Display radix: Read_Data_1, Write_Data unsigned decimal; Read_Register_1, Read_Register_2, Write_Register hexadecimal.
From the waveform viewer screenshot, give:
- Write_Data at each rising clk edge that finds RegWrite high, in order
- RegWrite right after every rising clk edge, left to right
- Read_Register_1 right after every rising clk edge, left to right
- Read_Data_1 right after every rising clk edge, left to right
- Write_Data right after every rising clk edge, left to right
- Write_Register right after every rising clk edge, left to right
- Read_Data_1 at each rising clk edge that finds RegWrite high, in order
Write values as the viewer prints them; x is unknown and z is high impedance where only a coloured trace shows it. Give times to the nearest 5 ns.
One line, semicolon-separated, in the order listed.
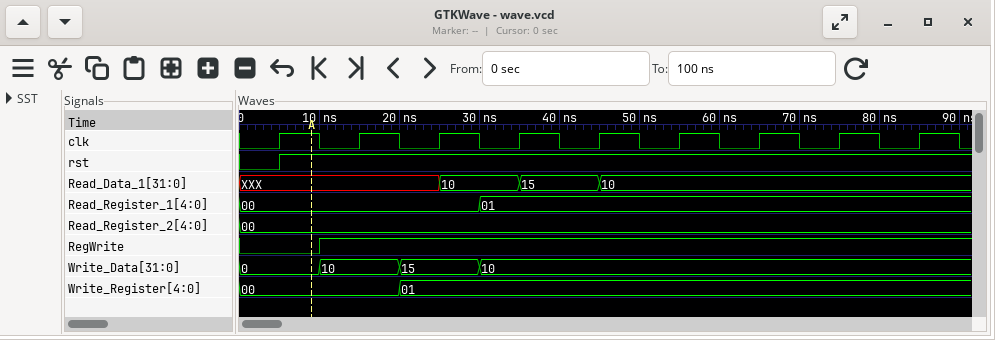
10, 15, 10, 10, 10, 10, 10, 10; 0 1 1 1 1 1 1 1 1; 00, 00, 00, 01, 01, 01, 01, 01, 01; XXX, XXX, 10, 15, 10, 10, 10, 10, 10; 0, 10, 15, 10, 10, 10, 10, 10, 10; 00, 00, 01, 01, 01, 01, 01, 01, 01; XXX, XXX, 10, 15, 10, 10, 10, 10
